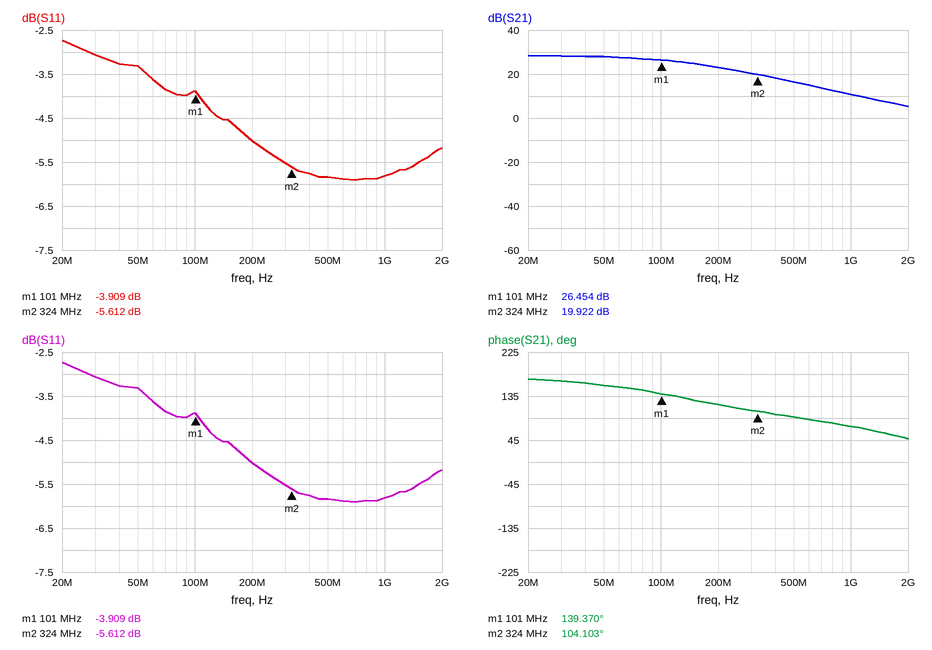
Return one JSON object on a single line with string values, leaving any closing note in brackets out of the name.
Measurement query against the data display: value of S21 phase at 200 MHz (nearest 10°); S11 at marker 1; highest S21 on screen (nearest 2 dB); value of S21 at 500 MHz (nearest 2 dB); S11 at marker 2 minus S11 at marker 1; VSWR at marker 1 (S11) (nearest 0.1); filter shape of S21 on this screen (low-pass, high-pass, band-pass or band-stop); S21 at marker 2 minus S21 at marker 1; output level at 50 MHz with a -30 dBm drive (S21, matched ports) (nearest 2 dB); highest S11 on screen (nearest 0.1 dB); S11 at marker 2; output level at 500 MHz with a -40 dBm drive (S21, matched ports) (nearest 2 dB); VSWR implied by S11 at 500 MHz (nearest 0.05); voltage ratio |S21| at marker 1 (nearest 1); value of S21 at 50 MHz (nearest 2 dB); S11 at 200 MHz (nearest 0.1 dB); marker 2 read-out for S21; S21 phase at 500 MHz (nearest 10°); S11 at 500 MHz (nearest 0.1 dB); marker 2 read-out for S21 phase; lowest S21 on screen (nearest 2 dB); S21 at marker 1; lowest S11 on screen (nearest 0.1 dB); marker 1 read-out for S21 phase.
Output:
{"value of S21 phase at 200 MHz": "120°", "S11 at marker 1": "-3.909 dB", "highest S21 on screen": "28 dB", "value of S21 at 500 MHz": "16 dB", "S11 at marker 2 minus S11 at marker 1": "-1.703 dB", "VSWR at marker 1 (S11)": "4.5", "filter shape of S21 on this screen": "low-pass", "S21 at marker 2 minus S21 at marker 1": "-6.532 dB", "output level at 50 MHz with a -30 dBm drive (S21, matched ports)": "-2 dBm", "highest S11 on screen": "-2.7 dB", "S11 at marker 2": "-5.612 dB", "output level at 500 MHz with a -40 dBm drive (S21, matched ports)": "-24 dBm", "VSWR implied by S11 at 500 MHz": "3.10", "voltage ratio |S21| at marker 1": "21", "value of S21 at 50 MHz": "28 dB", "S11 at 200 MHz": "-5.0 dB", "marker 2 read-out for S21": "19.922 dB", "S21 phase at 500 MHz": "90°", "S11 at 500 MHz": "-5.8 dB", "marker 2 read-out for S21 phase": "104.103°", "lowest S21 on screen": "6 dB", "S21 at marker 1": "26.454 dB", "lowest S11 on screen": "-5.9 dB", "marker 1 read-out for S21 phase": "139.370°"}
